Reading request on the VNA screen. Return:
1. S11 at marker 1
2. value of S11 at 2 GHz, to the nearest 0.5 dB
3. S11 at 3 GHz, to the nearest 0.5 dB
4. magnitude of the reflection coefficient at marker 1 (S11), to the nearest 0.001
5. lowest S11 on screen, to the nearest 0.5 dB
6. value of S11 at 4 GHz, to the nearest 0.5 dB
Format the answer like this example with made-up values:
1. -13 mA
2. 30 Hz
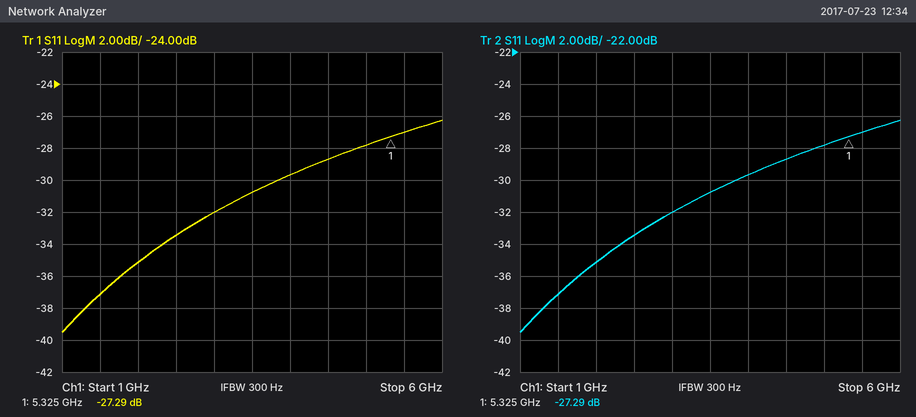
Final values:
1. -27.29 dB
2. -35.0 dB
3. -32.0 dB
4. 0.043
5. -39.5 dB
6. -29.5 dB
